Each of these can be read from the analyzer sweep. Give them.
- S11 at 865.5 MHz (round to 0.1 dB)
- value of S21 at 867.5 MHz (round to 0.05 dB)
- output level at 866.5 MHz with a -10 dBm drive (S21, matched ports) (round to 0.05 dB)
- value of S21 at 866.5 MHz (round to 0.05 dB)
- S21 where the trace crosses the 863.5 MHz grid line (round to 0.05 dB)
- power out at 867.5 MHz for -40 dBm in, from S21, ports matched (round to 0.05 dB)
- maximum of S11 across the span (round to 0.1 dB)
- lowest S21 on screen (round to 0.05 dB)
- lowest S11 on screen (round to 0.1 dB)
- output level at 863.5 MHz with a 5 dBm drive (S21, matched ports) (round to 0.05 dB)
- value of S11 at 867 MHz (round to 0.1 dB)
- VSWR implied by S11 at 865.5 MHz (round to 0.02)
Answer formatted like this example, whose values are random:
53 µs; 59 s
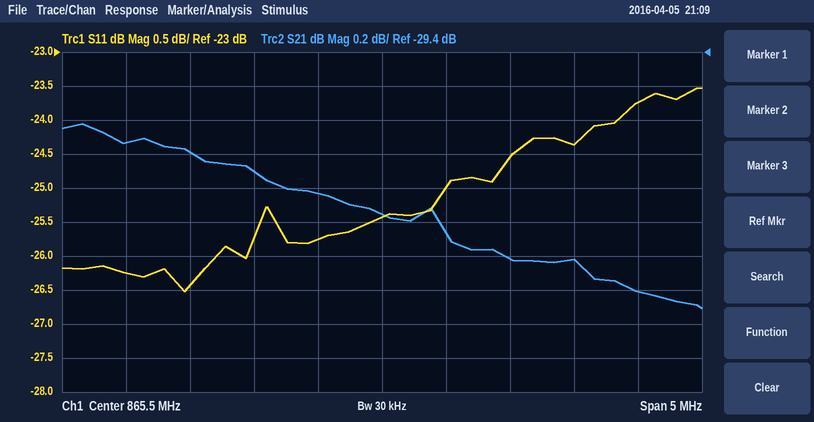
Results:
-25.4 dB; -30.80 dB; -40.60 dBm; -30.60 dB; -29.95 dB; -70.80 dBm; -23.5 dB; -30.90 dB; -26.5 dB; -24.95 dBm; -24.4 dB; 1.12
